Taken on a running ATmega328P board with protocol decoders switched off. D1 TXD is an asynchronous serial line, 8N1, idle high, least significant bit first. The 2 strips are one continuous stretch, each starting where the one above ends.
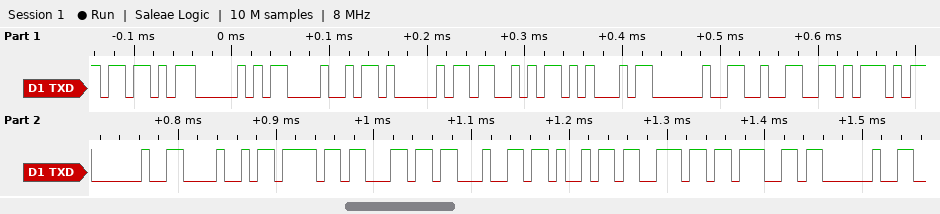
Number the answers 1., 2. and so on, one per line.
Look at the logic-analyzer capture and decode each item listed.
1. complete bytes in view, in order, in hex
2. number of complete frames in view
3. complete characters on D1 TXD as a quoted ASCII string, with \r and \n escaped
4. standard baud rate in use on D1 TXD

1. 5B 50 48 41 53 45 20 32 5D 20 48 6F 6C 64 69 6E 67 20
2. 18
3. "[PHASE 2] Holding "
4. 115200 baud
